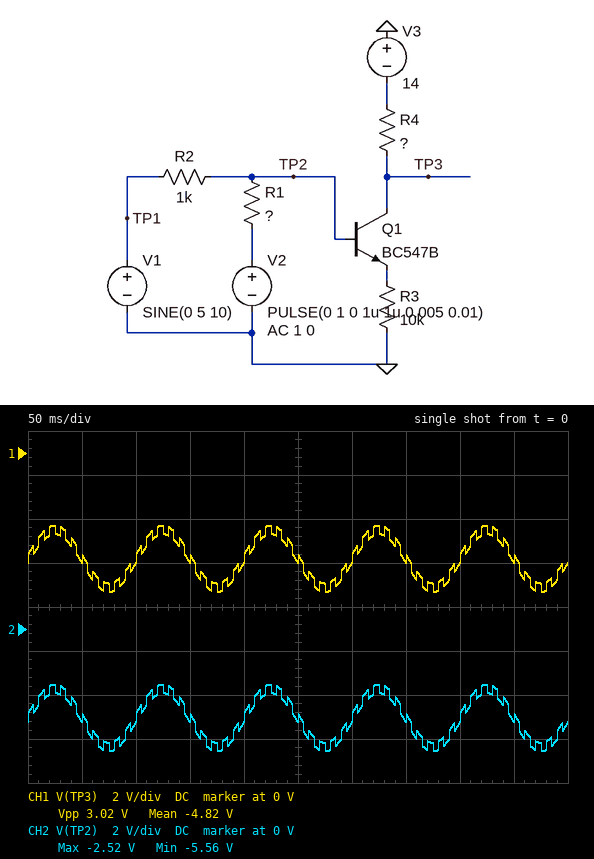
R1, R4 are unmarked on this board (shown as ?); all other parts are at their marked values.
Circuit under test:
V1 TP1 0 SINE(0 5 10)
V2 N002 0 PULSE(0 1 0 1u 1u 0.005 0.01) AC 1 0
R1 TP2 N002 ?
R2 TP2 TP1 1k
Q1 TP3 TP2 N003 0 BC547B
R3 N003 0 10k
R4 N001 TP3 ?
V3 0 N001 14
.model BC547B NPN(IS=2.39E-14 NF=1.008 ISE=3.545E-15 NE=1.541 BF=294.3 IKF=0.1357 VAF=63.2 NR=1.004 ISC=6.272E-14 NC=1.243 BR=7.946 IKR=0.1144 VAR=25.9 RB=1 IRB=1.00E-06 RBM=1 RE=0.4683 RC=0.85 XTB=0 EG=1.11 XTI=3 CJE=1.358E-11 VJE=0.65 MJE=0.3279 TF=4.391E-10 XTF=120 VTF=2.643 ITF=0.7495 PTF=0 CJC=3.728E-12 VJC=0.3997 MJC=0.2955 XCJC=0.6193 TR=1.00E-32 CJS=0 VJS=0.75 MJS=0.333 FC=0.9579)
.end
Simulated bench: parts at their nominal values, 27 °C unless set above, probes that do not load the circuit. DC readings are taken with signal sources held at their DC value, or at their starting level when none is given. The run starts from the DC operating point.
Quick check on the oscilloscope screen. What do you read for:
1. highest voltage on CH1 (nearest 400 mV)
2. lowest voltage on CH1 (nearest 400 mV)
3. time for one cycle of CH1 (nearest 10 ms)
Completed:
-3.2 V
-6.4 V
100 ms
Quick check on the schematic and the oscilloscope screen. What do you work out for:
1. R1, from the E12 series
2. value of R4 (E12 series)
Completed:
680 Ω
820 Ω
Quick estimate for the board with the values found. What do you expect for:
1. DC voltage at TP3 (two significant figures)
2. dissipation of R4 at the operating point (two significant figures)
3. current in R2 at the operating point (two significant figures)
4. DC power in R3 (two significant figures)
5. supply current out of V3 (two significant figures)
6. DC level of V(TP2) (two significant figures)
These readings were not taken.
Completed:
-5.0 V
99 mW
4.2 mA
2.5 mW
11 mA
-4.2 V
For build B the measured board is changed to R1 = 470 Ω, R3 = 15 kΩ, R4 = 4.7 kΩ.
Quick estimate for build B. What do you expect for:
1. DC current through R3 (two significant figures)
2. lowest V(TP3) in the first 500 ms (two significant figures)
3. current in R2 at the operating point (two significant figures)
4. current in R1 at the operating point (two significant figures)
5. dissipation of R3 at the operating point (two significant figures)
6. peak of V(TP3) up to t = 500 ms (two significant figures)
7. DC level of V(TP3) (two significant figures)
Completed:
100 µA
-3.0 V
820 µA
1.7 mA
160 µW
560 mV
-1.5 V
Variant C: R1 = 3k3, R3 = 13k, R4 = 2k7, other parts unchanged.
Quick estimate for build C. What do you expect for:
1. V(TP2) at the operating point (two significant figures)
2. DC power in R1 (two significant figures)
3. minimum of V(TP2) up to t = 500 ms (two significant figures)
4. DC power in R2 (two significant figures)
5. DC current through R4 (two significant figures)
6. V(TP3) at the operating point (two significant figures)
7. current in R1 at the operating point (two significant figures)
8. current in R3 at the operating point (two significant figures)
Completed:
-2.8 V
2.3 mW
-5.6 V
7.7 mW
3.9 mA
-3.5 V
840 µA
270 µA
